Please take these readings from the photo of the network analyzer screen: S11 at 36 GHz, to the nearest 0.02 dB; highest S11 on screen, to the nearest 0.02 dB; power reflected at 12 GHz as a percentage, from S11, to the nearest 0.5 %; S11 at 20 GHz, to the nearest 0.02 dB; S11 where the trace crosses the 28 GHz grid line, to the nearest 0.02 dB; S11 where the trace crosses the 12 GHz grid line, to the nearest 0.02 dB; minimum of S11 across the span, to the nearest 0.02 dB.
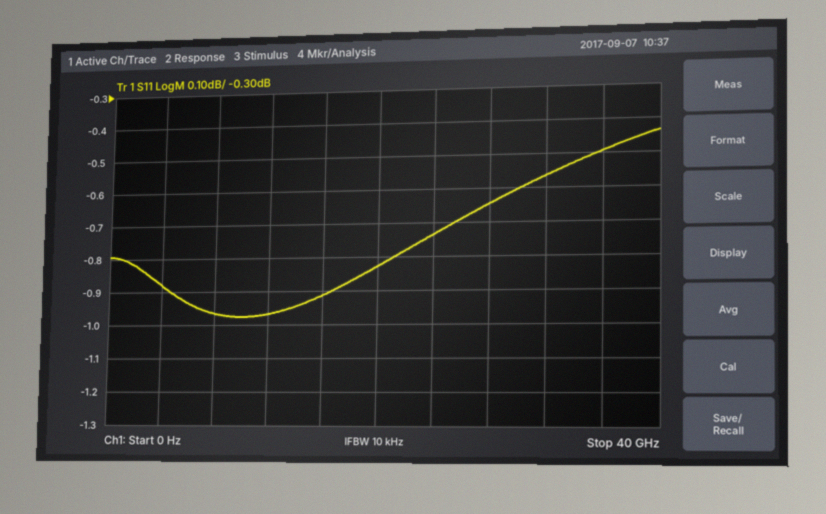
-0.50 dB
-0.44 dB
80.0 %
-0.82 dB
-0.64 dB
-0.96 dB
-0.98 dB
